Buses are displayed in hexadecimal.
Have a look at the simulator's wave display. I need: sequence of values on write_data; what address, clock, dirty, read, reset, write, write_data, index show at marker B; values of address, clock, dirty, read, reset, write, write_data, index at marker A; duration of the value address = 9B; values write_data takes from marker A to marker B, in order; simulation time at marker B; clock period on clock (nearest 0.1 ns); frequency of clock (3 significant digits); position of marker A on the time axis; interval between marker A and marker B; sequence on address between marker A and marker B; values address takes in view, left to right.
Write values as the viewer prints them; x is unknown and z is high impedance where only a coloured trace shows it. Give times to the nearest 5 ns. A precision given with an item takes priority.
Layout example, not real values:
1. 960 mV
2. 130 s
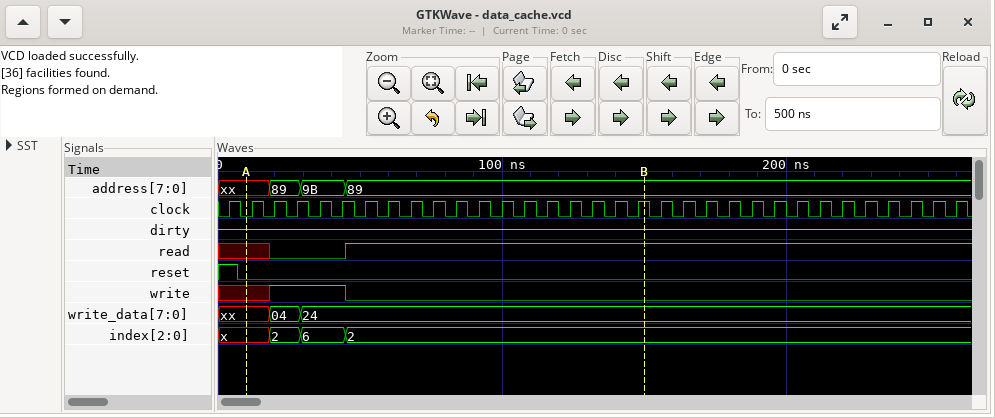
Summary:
1. xx, 04, 24
2. address=89, clock=1, dirty=z, read=1, reset=0, write=0, write_data=24, index=2
3. address=xx, clock=0, dirty=z, read=x, reset=0, write=x, write_data=xx, index=x
4. 15 ns
5. xx, 04, 24
6. 150 ns
7. 8 ns
8. 125 MHz
9. 10 ns
10. 140 ns
11. xx, 89, 9B, 89
12. xx, 89, 9B, 89
